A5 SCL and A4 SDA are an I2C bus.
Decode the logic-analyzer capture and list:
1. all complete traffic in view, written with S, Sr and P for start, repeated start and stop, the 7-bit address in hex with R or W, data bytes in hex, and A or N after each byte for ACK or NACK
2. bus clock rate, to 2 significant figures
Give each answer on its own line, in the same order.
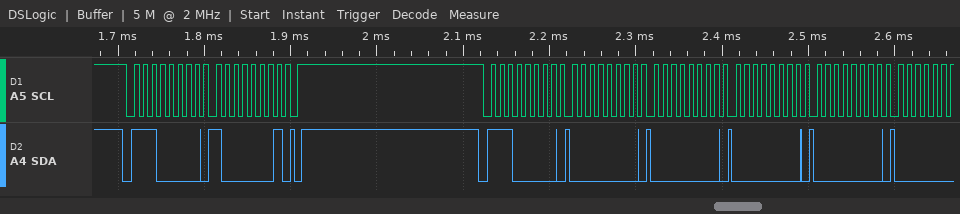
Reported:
S 70W A 81 A P S 70W A 00 A 00 A 00 A 00 A
100 kHz
